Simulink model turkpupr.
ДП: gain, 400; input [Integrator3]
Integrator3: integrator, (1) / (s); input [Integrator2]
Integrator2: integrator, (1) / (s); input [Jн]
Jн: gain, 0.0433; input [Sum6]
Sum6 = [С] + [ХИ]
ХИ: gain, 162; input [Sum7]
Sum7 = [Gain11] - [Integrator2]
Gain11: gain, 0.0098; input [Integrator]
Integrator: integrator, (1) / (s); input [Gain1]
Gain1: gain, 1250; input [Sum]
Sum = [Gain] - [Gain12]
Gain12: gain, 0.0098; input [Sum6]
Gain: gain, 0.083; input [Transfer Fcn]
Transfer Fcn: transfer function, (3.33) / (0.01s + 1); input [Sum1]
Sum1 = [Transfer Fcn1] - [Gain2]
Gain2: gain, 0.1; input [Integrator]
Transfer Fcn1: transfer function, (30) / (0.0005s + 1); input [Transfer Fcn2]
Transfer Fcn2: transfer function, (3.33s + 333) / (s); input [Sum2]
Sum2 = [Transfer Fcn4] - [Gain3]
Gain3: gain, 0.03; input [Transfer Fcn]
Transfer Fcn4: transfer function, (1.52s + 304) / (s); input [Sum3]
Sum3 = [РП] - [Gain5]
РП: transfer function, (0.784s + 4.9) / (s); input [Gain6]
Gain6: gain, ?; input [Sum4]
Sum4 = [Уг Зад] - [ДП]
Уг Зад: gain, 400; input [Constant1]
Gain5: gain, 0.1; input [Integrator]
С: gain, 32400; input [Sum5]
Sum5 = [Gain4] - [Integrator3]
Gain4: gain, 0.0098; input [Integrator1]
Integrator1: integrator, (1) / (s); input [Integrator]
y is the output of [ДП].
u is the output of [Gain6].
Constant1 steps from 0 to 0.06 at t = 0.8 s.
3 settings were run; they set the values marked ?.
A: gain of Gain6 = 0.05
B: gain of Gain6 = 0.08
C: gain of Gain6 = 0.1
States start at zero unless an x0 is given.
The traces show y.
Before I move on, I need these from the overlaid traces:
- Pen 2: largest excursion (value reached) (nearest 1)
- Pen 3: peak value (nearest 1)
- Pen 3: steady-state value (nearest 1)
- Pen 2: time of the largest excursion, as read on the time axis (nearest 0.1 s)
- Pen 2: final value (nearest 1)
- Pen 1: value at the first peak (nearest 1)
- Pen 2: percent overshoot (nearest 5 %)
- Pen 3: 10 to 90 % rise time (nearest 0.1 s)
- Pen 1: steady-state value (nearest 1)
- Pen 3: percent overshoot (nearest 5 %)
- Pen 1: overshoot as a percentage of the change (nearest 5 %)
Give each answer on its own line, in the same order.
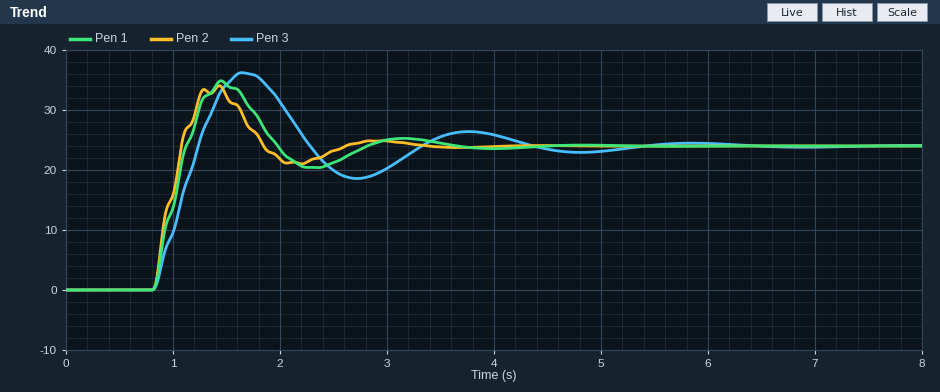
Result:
34
36
24
1.4 s
24
35
40 %
0.3 s
24
50 %
45 %
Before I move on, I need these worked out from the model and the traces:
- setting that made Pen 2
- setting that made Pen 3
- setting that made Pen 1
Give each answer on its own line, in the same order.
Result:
C
A
B
